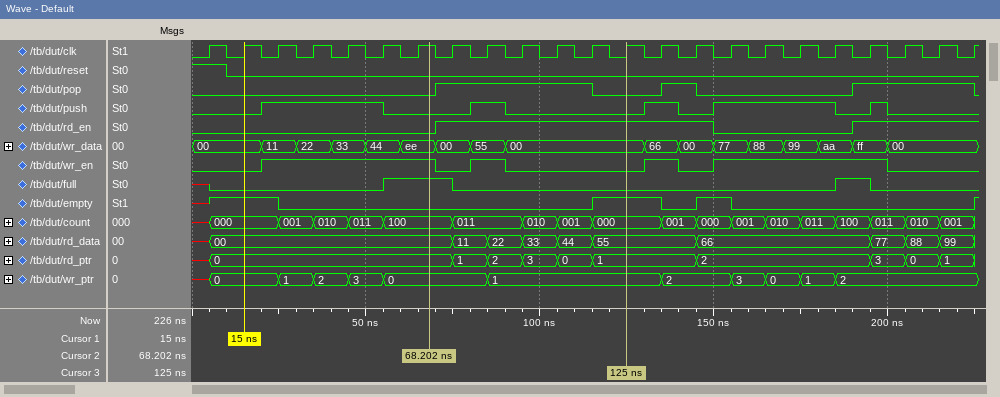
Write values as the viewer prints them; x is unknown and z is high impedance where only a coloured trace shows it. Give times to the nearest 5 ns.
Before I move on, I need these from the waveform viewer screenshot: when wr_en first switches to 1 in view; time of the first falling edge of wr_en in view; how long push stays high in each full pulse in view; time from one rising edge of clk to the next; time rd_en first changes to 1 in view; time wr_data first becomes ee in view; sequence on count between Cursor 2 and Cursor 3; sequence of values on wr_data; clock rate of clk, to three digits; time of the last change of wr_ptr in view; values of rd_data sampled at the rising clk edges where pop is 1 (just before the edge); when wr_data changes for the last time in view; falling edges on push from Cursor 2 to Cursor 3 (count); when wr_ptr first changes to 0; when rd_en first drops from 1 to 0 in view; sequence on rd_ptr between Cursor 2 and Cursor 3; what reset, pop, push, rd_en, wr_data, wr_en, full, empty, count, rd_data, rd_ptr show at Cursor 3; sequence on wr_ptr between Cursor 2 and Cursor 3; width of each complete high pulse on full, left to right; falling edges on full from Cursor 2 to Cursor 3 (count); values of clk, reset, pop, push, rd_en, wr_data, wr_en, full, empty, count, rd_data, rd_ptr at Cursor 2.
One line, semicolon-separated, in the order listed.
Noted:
20 ns; 70 ns; 35 ns, 10 ns, 10 ns, 35 ns, 5 ns; 10 ns; 70 ns; 60 ns; 100, 011, 010, 001, 000; 00, 11, 22, 33, 44, ee, 00, 55, 00, 66, 00, 77, 88, 99, aa, ff, 00; 100 MHz; 185 ns; 00, 11, 22, 33, 44, 55, 66, 77, 88, 99; 200 ns; 1; 5 ns; 150 ns; 0, 1, 2, 3, 0, 1; reset=0, pop=0, push=0, rd_en=1, wr_data=00, wr_en=0, full=0, empty=1, count=000, rd_data=55, rd_ptr=1; 0, 1; 20 ns, 10 ns; 1; clk=1, reset=0, pop=0, push=0, rd_en=0, wr_data=ee, wr_en=1, full=1, empty=0, count=100, rd_data=00, rd_ptr=0
